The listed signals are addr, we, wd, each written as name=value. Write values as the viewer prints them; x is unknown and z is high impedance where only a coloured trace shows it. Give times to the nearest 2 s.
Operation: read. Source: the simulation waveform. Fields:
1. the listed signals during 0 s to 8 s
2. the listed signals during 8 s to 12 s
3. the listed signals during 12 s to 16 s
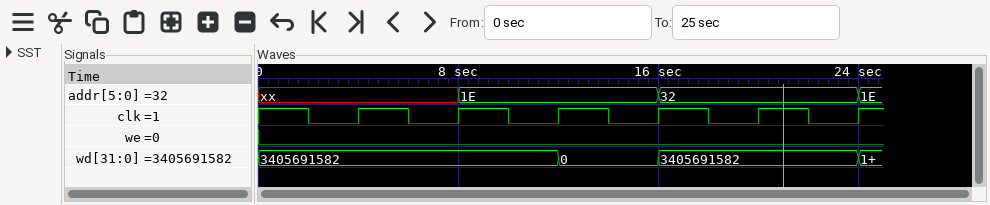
addr=xx, we=0, wd=3405691582
addr=1E, we=0, wd=3405691582
addr=1E, we=0, wd=0
